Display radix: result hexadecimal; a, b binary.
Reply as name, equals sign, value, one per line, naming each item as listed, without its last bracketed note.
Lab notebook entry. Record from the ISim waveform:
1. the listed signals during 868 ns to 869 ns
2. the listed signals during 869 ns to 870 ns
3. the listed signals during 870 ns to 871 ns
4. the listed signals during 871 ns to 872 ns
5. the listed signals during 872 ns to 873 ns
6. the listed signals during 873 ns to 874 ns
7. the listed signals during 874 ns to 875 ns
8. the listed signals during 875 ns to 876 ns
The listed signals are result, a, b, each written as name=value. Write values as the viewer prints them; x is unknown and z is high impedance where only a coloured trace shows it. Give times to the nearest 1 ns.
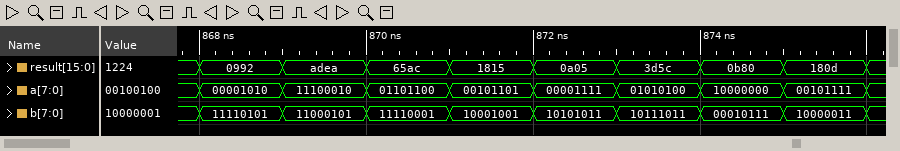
the listed signals during 868 ns to 869 ns = result=0992, a=00001010, b=11110101
the listed signals during 869 ns to 870 ns = result=adea, a=11100010, b=11000101
the listed signals during 870 ns to 871 ns = result=65ac, a=01101100, b=11110001
the listed signals during 871 ns to 872 ns = result=1815, a=00101101, b=10001001
the listed signals during 872 ns to 873 ns = result=0a05, a=00001111, b=10101011
the listed signals during 873 ns to 874 ns = result=3d5c, a=01010100, b=10111011
the listed signals during 874 ns to 875 ns = result=0b80, a=10000000, b=00010111
the listed signals during 875 ns to 876 ns = result=180d, a=00101111, b=10000011
